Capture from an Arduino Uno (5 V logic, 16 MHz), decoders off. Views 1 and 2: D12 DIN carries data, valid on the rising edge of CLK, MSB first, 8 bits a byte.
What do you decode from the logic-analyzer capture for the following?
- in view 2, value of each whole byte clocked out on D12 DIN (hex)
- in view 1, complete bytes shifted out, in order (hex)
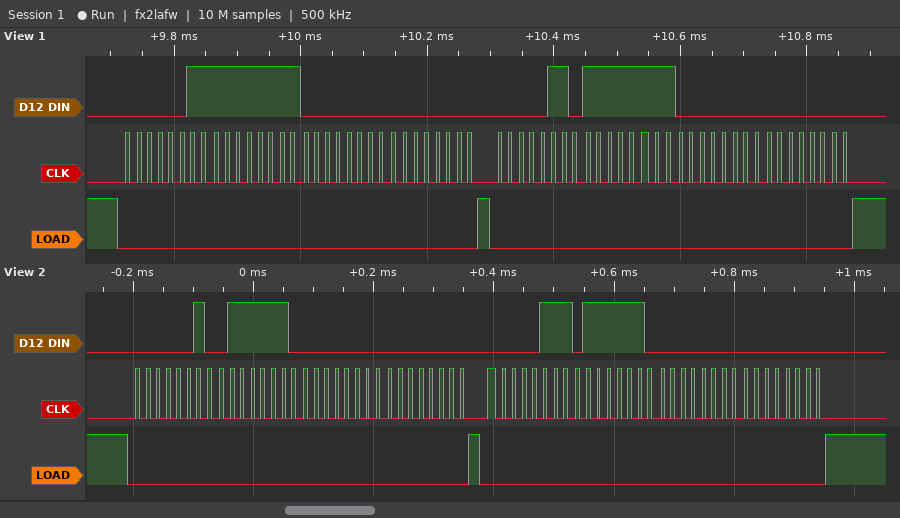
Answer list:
0x02 0x7E 0x00 0x00 0x07 0x7E 0x00 0x00
03 FF 00 00 06 FF 00 00
